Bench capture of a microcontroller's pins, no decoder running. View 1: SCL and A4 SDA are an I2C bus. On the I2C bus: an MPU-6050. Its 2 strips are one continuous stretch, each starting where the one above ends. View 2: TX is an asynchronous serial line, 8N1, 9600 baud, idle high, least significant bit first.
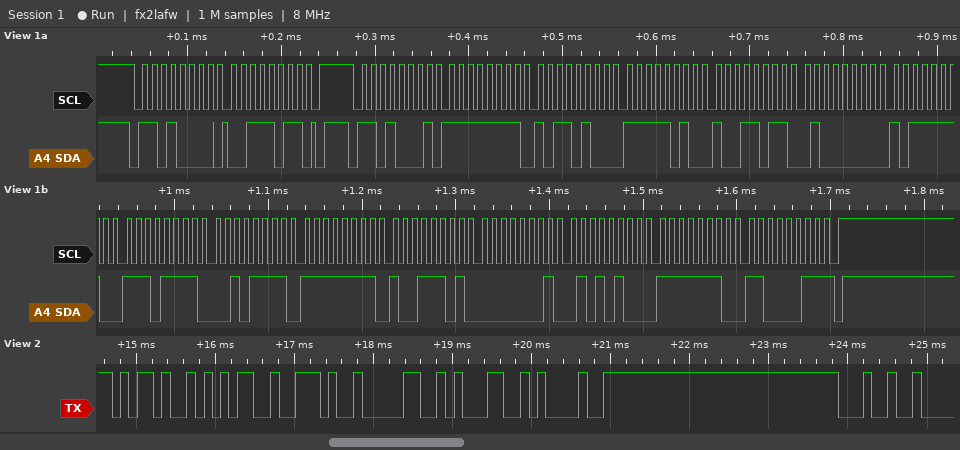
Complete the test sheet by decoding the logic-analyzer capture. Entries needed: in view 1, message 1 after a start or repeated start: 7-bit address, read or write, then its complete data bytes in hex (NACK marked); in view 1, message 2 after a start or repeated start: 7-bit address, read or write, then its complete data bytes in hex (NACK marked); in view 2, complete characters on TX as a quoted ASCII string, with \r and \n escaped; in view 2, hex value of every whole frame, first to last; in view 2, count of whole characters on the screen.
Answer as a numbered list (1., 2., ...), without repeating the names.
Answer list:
1. 0x68 write: 3B
2. 0x68 read: FF B4 FA 9B 40 BE EF 2F FF 9D 01 54 FE C3 NACK
3. "-5.01!$"
4. 2D 35 2E 30 31 21 24
5. 7
